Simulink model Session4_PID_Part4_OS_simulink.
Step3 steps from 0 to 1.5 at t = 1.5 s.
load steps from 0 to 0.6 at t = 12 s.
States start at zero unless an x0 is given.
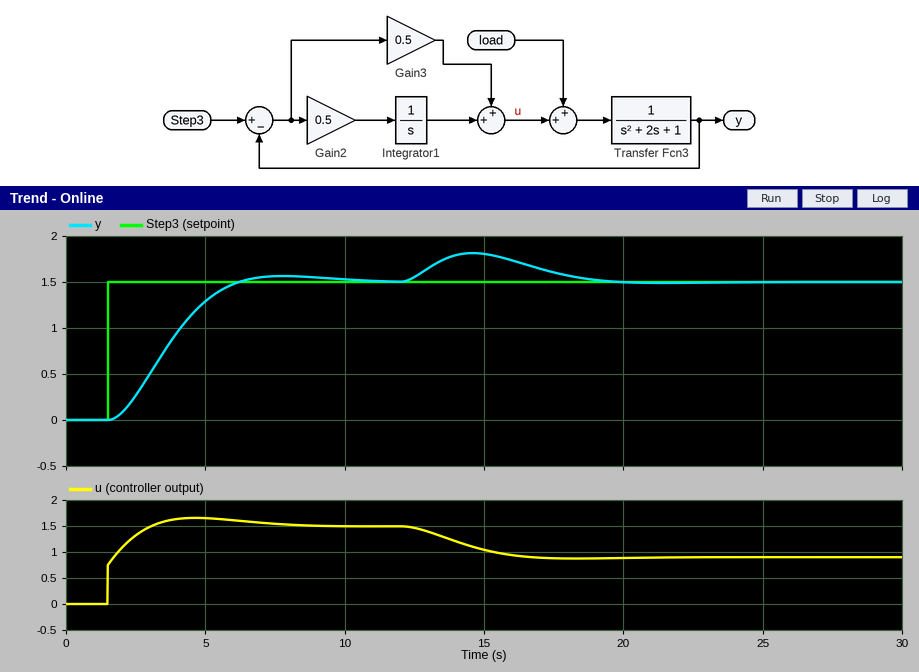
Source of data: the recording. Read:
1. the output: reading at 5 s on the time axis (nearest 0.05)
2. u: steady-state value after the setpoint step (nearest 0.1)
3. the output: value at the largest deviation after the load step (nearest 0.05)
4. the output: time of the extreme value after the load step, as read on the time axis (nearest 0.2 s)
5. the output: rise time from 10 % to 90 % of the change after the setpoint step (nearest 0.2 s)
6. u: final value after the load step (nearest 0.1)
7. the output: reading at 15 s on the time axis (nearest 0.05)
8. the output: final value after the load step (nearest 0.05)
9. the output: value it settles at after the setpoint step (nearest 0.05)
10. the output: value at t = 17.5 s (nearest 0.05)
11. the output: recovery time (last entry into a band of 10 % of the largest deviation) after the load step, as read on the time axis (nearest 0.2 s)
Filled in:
1.30
1.5
1.80
14.6 s
3.0 s
0.9
1.80
1.50
1.50
1.60
18.8 s
